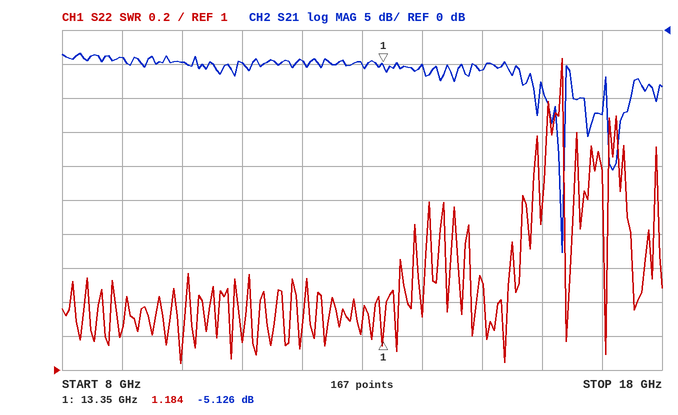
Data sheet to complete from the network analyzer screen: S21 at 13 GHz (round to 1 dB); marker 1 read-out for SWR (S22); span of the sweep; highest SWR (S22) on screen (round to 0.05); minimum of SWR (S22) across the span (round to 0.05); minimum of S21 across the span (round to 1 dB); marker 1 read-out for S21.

-5 dB
1.184
10 GHz
2.85
1.05
-33 dB
-5.126 dB
